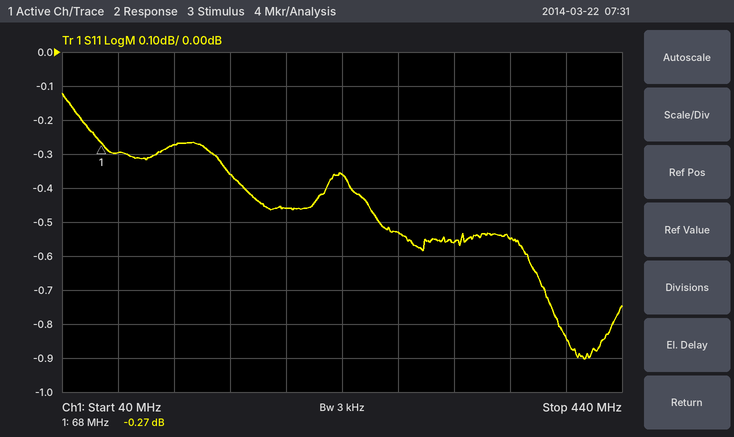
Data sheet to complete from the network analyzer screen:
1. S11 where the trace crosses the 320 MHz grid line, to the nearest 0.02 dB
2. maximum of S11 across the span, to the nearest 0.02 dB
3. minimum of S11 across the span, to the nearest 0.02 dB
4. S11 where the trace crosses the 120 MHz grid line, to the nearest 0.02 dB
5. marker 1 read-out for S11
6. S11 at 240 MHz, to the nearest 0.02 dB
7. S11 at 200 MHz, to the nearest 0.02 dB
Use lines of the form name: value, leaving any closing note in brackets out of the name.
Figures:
S11 where the trace crosses the 320 MHz grid line, to the nearest 0.02 dB: -0.56 dB
maximum of S11 across the span, to the nearest 0.02 dB: -0.12 dB
minimum of S11 across the span, to the nearest 0.02 dB: -0.90 dB
S11 where the trace crosses the 120 MHz grid line, to the nearest 0.02 dB: -0.28 dB
marker 1 read-out for S11: -0.27 dB
S11 at 240 MHz, to the nearest 0.02 dB: -0.36 dB
S11 at 200 MHz, to the nearest 0.02 dB: -0.46 dB
